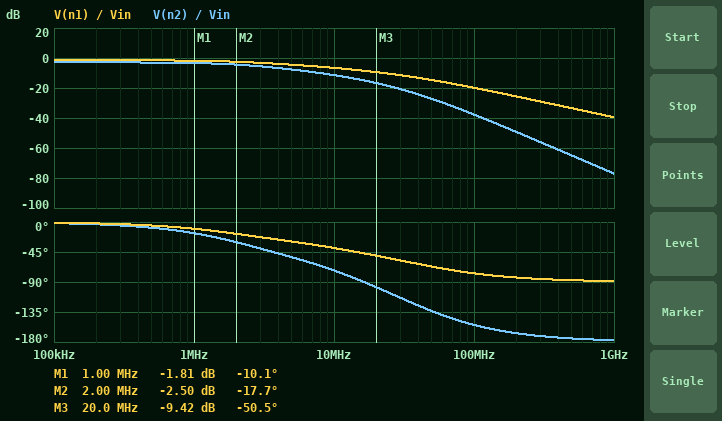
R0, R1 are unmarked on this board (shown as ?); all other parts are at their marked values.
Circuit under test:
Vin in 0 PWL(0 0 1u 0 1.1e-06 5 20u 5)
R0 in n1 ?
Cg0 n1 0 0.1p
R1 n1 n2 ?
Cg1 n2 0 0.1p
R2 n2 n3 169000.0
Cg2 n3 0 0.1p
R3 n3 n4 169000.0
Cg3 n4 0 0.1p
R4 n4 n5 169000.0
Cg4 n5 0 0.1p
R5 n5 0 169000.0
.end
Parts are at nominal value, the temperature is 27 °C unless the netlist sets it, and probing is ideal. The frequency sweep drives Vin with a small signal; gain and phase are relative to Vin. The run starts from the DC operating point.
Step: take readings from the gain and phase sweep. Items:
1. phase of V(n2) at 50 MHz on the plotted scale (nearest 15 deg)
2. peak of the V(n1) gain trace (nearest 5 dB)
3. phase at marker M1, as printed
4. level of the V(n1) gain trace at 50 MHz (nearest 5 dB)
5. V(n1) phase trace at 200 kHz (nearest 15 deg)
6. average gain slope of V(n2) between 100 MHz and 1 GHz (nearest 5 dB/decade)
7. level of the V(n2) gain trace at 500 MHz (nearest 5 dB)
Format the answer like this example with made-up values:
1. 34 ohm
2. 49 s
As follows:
1. -135 deg
2. 0 dB
3. -10.1 deg
4. -15 dB
5. 0 deg
6. -40 dB/decade
7. -65 dB
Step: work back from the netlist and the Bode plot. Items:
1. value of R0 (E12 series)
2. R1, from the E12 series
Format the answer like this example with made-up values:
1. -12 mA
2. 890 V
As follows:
1. 150 kΩ
2. 120 kΩ
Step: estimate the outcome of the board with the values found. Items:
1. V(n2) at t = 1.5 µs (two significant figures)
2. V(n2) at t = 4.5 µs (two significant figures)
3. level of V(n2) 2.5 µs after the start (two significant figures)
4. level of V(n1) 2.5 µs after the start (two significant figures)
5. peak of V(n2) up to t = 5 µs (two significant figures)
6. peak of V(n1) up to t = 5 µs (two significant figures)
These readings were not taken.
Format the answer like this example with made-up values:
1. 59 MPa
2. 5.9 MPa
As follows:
1. 3.6 V
2. 3.6 V
3. 3.6 V
4. 4.2 V
5. 3.6 V
6. 4.2 V
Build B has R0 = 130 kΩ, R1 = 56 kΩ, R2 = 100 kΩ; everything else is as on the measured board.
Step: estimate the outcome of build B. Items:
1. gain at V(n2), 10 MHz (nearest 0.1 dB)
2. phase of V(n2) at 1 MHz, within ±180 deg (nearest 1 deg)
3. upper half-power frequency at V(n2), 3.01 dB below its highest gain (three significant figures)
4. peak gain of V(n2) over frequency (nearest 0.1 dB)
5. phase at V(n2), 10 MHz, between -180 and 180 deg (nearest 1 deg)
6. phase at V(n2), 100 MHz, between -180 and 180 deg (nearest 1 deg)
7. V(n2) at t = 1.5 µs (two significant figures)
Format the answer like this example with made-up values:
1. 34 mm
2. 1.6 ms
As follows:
1. -9.9 dB
2. -14 deg
3. 3.85 MHz
4. -2.3 dB
5. -63 deg
6. -137 deg
7. 3.8 V
